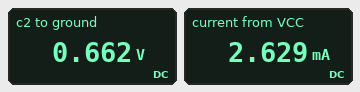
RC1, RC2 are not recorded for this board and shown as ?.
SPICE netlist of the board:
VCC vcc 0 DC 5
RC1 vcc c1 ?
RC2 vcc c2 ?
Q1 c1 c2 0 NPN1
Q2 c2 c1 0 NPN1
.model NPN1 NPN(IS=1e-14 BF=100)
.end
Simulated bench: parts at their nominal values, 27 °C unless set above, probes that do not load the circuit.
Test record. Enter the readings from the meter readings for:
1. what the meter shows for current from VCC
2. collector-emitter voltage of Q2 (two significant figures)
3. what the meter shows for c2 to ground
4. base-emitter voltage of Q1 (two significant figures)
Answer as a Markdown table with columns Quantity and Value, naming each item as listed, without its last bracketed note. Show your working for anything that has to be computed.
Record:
| Quantity | Value |
|---|---|
| what the meter shows for current from VCC | 2.629 mA |
| collector-emitter voltage of Q2 | 662 mV = 660 mV |
| what the meter shows for c2 to ground | 0.662 V |
| base-emitter voltage of Q1 | 662 mV = 660 mV |
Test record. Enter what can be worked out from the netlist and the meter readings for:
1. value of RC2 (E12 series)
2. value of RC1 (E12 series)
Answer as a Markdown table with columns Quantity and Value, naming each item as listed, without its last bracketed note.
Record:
| Quantity | Value |
|---|---|
| value of RC2 | 3.3 kΩ |
| value of RC1 | 3.3 kΩ |
